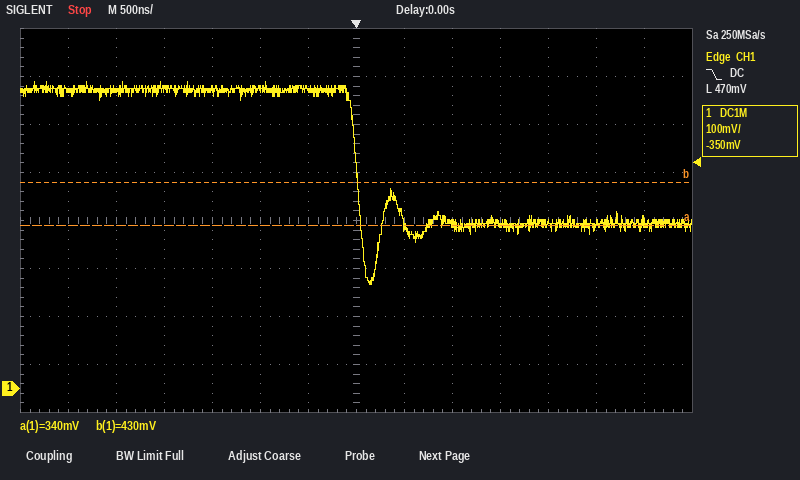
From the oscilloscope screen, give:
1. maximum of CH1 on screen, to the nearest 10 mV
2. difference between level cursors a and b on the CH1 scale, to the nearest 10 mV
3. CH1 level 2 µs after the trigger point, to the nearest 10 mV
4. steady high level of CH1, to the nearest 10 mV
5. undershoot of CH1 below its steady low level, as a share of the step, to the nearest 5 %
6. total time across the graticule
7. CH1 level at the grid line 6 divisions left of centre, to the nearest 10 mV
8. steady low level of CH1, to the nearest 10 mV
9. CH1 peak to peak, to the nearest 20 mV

640 mV
90 mV
340 mV
620 mV
45 %
7 µs
620 mV
340 mV
420 mV
